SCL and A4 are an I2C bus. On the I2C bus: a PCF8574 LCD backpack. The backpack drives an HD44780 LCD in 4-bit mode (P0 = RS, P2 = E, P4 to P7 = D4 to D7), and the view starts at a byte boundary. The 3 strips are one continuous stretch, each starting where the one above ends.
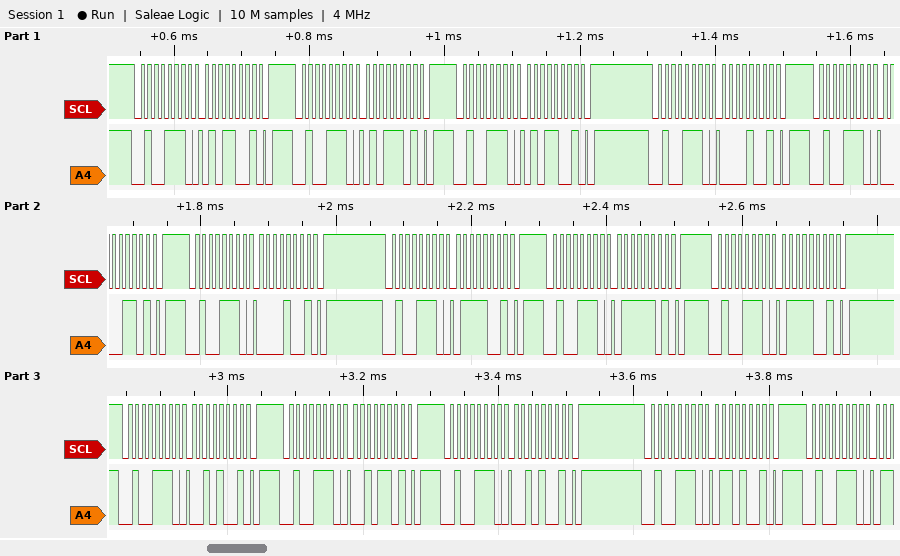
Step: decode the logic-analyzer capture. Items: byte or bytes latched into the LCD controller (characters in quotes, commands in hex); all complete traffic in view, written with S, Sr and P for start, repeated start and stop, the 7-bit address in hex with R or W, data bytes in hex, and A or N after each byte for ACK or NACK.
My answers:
'P' 'r'
S 27W A 59 A P S 27W A 5D A P S 27W A 59 A P S 27W A 09 A P S 27W A 0D A P S 27W A 09 A P S 27W A 79 A P S 27W A 7D A P S 27W A 79 A P S 27W A 29 A P S 27W A 2D A P S 27W A 29 A P S 27W A 69 A P S 27W A
